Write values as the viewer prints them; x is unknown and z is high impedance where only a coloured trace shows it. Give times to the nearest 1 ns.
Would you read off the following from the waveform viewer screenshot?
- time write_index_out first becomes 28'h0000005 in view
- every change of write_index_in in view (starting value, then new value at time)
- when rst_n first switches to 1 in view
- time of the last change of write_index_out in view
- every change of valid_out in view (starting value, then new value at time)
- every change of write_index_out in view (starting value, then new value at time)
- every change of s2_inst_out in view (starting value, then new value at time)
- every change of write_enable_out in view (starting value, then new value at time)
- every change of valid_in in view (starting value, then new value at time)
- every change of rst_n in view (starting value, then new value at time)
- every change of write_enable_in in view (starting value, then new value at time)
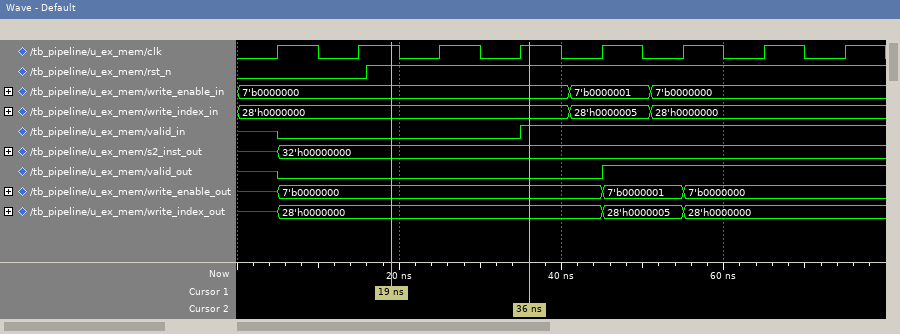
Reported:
45 ns
28'h0000000, 28'h0000005 at 41 ns, 28'h0000000 at 51 ns
16 ns
55 ns
x, 0 at 5 ns, 1 at 45 ns
x, 28'h0000000 at 5 ns, 28'h0000005 at 45 ns, 28'h0000000 at 55 ns
x, 32'h00000000 at 5 ns
x, 7'b0000000 at 5 ns, 7'b0000001 at 45 ns, 7'b0000000 at 55 ns
x, 0 at 5 ns, 1 at 35 ns
0, 1 at 16 ns
7'b0000000, 7'b0000001 at 41 ns, 7'b0000000 at 51 ns
